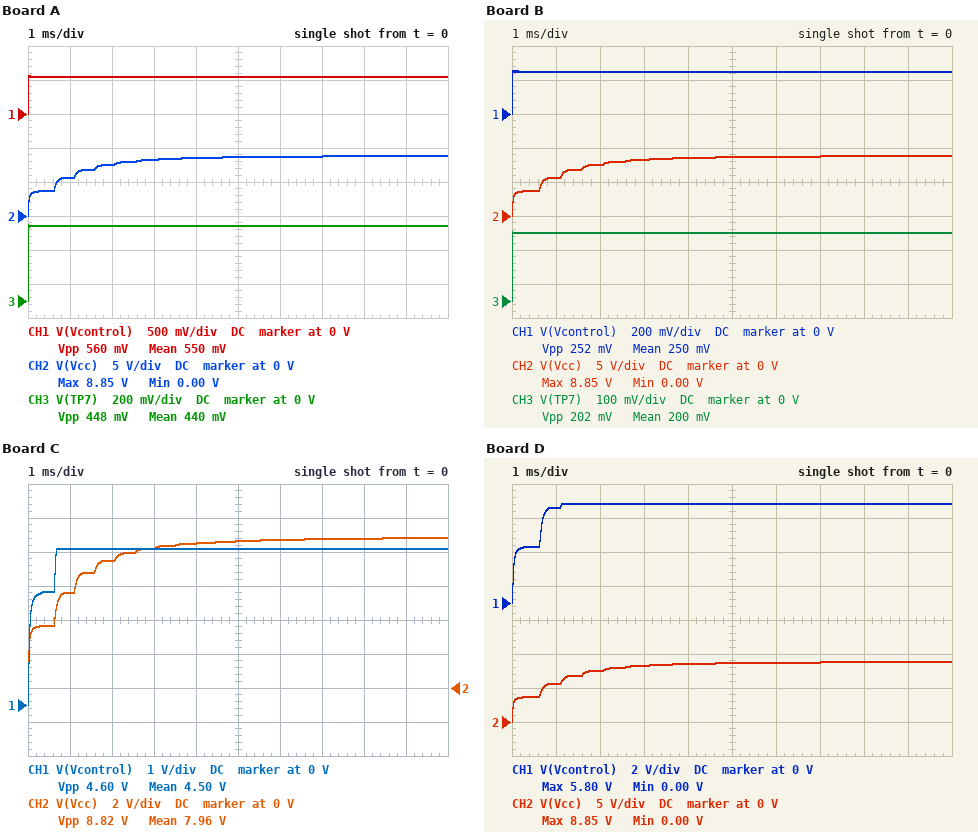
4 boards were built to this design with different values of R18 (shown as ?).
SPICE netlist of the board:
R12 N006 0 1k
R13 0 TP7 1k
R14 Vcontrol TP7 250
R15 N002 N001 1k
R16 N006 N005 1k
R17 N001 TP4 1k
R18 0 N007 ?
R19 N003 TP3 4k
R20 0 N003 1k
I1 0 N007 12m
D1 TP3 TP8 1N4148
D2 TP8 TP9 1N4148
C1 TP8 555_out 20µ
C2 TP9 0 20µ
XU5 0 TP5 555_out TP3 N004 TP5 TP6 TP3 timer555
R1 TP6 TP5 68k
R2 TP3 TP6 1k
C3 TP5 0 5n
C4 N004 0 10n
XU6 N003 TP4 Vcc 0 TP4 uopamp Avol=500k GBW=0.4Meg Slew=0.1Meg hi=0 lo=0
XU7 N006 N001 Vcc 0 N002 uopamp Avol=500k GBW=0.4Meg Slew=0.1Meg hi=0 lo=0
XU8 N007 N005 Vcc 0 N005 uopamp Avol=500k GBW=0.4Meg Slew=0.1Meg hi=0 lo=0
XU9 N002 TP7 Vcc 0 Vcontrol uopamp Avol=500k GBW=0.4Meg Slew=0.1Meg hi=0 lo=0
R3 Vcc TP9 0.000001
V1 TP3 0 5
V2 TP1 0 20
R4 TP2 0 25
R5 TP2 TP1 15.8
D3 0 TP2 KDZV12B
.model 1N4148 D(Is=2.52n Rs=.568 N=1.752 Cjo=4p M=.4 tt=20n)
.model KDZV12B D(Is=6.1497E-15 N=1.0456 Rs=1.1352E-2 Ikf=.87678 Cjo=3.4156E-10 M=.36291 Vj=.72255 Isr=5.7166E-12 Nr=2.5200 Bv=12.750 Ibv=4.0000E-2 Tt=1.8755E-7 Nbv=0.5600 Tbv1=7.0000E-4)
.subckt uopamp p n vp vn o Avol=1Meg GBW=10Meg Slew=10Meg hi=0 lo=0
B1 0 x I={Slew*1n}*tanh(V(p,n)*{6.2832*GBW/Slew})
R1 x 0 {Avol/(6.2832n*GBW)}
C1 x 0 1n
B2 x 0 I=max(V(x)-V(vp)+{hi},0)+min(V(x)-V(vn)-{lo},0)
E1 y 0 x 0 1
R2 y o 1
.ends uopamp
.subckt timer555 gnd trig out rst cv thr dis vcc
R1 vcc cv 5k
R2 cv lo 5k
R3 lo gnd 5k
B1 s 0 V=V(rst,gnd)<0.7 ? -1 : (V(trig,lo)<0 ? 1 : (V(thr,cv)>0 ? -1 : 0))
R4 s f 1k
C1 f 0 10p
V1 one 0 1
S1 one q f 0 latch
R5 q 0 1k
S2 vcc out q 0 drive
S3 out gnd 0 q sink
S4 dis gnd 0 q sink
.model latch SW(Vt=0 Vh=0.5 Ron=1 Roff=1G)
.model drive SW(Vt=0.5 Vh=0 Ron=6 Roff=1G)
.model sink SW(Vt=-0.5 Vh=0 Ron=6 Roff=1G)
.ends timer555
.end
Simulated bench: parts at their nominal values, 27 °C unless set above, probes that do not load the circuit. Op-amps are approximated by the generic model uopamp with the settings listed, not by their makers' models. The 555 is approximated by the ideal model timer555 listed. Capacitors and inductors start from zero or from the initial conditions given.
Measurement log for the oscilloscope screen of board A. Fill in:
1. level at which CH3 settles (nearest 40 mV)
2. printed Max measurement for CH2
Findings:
440 mV
8.85 V
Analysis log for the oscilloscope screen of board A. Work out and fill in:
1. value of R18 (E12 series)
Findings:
120 Ω
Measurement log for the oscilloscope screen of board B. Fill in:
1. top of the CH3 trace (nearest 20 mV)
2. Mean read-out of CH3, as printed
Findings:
200 mV
200 mV
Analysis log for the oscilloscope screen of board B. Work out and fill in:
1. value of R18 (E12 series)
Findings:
100 Ω
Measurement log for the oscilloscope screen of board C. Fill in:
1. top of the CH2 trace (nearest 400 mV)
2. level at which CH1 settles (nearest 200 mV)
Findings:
8.8 V
4.6 V
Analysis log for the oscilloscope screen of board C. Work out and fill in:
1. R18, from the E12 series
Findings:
390 Ω
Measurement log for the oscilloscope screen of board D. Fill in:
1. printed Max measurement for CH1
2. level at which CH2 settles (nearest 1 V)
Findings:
5.80 V
9 V
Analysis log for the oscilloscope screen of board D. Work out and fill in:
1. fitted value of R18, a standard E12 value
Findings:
470 Ω
